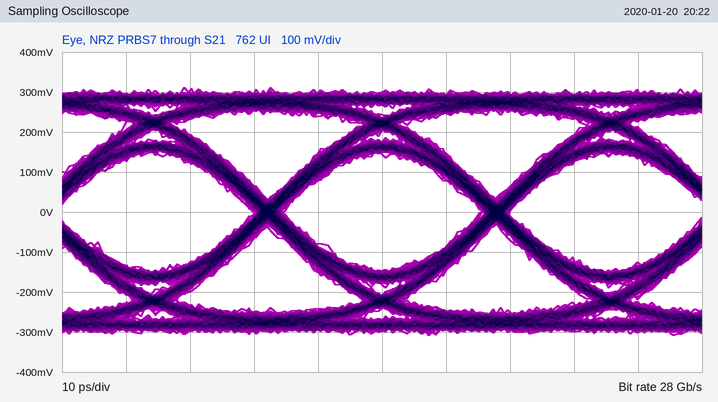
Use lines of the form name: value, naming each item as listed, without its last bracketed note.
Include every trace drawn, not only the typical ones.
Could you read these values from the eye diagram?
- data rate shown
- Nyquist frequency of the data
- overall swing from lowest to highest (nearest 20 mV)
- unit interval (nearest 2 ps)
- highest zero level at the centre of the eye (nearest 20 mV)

data rate shown: 28 Gb/s
Nyquist frequency of the data: 14 GHz
overall swing from lowest to highest: 620 mV
unit interval: 36 ps
highest zero level at the centre of the eye: -140 mV
